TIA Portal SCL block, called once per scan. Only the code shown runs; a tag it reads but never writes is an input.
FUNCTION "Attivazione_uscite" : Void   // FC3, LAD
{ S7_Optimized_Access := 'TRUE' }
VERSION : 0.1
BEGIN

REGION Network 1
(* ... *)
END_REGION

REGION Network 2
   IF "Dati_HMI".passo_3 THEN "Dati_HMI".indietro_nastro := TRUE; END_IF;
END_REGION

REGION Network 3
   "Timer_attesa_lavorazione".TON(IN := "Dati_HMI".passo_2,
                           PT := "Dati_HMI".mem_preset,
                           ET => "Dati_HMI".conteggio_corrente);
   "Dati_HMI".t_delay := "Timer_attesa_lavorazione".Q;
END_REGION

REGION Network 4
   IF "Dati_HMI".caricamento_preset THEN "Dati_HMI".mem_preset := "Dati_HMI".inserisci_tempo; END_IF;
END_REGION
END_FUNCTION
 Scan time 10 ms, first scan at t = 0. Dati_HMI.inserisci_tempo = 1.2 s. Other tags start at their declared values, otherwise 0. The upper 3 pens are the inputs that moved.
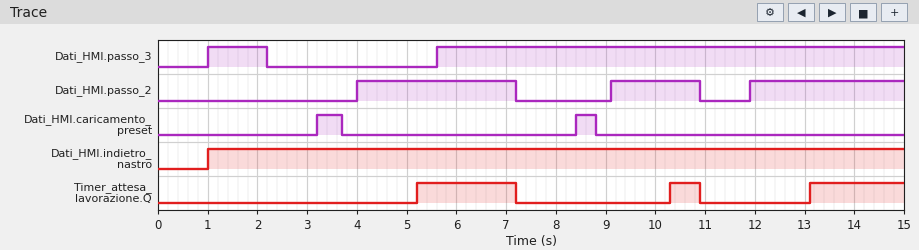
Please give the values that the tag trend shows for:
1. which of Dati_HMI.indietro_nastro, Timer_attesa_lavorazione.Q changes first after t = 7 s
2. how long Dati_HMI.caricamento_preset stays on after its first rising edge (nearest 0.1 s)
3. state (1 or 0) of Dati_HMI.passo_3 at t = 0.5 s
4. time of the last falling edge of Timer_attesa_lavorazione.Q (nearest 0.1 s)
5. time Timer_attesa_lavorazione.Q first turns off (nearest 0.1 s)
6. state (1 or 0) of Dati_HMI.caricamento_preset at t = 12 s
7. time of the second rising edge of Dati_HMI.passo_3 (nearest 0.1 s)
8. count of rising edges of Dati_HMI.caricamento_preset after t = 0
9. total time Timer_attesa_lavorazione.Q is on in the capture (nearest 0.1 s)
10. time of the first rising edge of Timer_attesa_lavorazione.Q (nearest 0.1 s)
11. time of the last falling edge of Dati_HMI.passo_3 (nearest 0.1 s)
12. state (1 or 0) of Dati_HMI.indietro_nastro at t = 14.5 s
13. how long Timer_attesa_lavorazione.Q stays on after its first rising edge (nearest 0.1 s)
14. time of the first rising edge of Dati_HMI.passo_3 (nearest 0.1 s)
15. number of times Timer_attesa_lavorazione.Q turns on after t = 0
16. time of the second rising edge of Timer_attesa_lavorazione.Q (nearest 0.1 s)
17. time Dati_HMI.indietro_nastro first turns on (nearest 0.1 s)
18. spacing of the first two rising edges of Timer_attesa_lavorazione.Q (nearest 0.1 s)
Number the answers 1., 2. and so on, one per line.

1. Timer_attesa_lavorazione.Q
2. 0.5 s
3. 0
4. 10.9 s
5. 7.2 s
6. 0
7. 5.6 s
8. 2
9. 4.5 s
10. 5.2 s
11. 2.2 s
12. 1
13. 2.0 s
14. 1.0 s
15. 3
16. 10.3 s
17. 1.0 s
18. 5.1 s
